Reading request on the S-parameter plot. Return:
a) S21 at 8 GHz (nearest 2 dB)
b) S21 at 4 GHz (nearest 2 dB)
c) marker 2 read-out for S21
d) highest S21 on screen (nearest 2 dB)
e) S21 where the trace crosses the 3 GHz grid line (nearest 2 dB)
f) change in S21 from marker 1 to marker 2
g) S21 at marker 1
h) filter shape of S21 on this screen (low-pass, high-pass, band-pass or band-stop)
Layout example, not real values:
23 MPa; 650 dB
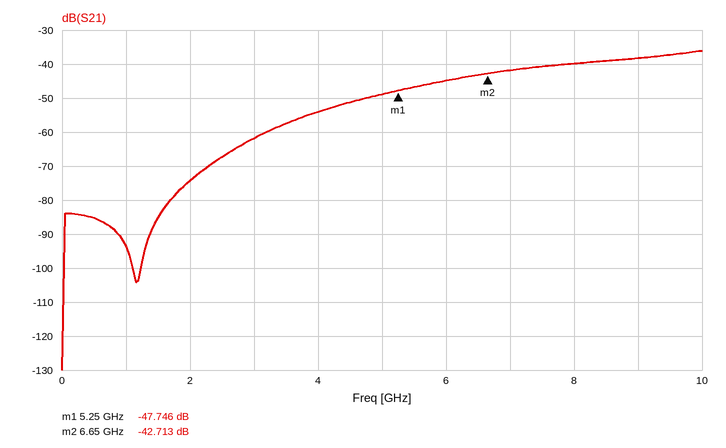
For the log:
-40 dB; -54 dB; -42.713 dB; -36 dB; -62 dB; 5.033 dB; -47.746 dB; high-pass
